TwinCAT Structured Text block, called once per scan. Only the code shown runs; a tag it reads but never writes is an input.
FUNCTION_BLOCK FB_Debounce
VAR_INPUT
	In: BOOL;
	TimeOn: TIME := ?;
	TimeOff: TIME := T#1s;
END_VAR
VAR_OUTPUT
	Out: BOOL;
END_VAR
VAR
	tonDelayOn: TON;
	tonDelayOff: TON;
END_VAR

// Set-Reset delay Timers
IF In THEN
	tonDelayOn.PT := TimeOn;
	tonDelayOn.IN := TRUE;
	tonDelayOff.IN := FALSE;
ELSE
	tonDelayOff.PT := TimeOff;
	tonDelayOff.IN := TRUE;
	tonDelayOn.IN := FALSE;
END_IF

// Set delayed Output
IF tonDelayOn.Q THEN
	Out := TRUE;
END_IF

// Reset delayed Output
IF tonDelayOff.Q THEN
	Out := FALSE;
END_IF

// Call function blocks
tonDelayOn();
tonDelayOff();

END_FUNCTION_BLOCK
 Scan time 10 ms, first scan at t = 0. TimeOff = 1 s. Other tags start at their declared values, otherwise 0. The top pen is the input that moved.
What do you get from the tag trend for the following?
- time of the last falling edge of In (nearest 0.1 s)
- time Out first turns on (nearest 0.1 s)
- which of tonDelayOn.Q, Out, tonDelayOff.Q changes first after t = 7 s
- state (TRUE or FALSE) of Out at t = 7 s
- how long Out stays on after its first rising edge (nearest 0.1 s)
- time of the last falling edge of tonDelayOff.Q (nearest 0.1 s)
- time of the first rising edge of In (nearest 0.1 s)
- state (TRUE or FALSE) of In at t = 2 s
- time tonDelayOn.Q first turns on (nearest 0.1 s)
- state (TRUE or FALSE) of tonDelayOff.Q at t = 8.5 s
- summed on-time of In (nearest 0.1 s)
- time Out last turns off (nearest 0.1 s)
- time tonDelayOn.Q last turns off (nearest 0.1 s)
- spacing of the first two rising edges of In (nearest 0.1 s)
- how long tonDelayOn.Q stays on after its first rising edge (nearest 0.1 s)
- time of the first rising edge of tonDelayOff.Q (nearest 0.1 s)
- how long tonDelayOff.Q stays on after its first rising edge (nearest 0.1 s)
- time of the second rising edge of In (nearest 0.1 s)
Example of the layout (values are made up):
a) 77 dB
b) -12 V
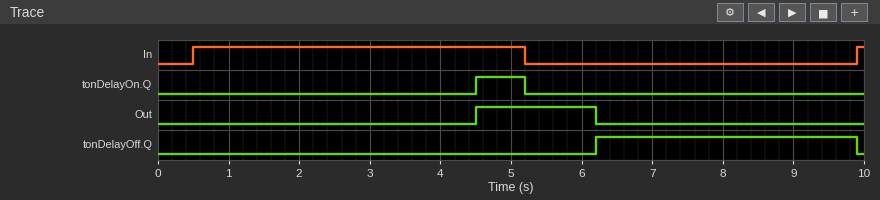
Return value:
a) 5.2 s
b) 4.5 s
c) tonDelayOff.Q
d) FALSE
e) 1.7 s
f) 9.9 s
g) 0.5 s
h) TRUE
i) 4.5 s
j) TRUE
k) 4.8 s
l) 6.2 s
m) 5.2 s
n) 9.4 s
o) 0.7 s
p) 6.2 s
q) 3.7 s
r) 9.9 s
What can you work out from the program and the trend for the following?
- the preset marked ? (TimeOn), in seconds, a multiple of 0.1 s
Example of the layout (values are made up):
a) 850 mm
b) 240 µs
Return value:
a) 4.0 s
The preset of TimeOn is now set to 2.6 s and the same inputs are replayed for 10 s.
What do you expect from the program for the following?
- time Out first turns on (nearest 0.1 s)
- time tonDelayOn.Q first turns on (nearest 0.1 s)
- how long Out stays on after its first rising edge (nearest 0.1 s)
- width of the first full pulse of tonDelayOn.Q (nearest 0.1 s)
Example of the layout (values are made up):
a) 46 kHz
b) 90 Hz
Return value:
a) 3.1 s
b) 3.1 s
c) 3.1 s
d) 2.1 s
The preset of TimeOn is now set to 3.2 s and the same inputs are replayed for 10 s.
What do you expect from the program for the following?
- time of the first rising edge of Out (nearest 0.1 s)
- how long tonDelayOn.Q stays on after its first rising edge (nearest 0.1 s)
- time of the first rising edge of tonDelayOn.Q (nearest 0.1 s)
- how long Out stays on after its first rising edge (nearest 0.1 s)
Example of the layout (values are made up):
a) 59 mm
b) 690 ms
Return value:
a) 3.7 s
b) 1.5 s
c) 3.7 s
d) 2.5 s
